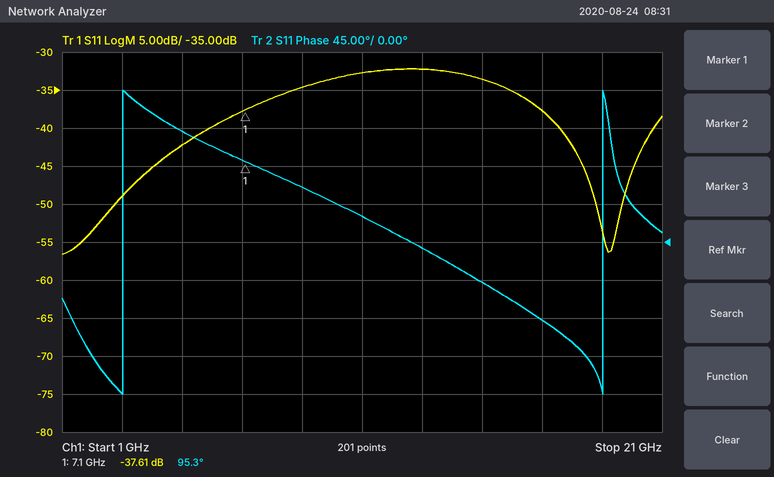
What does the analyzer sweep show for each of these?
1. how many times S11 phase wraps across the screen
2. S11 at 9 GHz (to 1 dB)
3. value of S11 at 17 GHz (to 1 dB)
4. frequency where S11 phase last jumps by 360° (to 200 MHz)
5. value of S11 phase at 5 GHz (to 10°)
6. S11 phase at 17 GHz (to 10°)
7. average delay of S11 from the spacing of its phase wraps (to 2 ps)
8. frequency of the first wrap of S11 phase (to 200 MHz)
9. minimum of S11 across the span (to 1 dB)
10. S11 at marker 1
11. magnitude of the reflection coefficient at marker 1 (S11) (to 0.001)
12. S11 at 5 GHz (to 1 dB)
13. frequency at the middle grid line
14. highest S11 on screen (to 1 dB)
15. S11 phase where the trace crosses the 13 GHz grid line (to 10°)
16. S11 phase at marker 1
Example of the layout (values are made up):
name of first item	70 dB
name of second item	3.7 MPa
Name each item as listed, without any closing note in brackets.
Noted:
how many times S11 phase wraps across the screen	2
S11 at 9 GHz	-35 dB
value of S11 at 17 GHz	-38 dB
frequency where S11 phase last jumps by 360°	19.0 GHz
value of S11 phase at 5 GHz	130°
S11 phase at 17 GHz	-90°
average delay of S11 from the spacing of its phase wraps	62 ps
frequency of the first wrap of S11 phase	3.0 GHz
minimum of S11 across the span	-57 dB
S11 at marker 1	-37.61 dB
magnitude of the reflection coefficient at marker 1 (S11)	0.013
S11 at 5 GHz	-42 dB
frequency at the middle grid line	11 GHz
highest S11 on screen	-32 dB
S11 phase where the trace crosses the 13 GHz grid line	-10°
S11 phase at marker 1	95.3°
